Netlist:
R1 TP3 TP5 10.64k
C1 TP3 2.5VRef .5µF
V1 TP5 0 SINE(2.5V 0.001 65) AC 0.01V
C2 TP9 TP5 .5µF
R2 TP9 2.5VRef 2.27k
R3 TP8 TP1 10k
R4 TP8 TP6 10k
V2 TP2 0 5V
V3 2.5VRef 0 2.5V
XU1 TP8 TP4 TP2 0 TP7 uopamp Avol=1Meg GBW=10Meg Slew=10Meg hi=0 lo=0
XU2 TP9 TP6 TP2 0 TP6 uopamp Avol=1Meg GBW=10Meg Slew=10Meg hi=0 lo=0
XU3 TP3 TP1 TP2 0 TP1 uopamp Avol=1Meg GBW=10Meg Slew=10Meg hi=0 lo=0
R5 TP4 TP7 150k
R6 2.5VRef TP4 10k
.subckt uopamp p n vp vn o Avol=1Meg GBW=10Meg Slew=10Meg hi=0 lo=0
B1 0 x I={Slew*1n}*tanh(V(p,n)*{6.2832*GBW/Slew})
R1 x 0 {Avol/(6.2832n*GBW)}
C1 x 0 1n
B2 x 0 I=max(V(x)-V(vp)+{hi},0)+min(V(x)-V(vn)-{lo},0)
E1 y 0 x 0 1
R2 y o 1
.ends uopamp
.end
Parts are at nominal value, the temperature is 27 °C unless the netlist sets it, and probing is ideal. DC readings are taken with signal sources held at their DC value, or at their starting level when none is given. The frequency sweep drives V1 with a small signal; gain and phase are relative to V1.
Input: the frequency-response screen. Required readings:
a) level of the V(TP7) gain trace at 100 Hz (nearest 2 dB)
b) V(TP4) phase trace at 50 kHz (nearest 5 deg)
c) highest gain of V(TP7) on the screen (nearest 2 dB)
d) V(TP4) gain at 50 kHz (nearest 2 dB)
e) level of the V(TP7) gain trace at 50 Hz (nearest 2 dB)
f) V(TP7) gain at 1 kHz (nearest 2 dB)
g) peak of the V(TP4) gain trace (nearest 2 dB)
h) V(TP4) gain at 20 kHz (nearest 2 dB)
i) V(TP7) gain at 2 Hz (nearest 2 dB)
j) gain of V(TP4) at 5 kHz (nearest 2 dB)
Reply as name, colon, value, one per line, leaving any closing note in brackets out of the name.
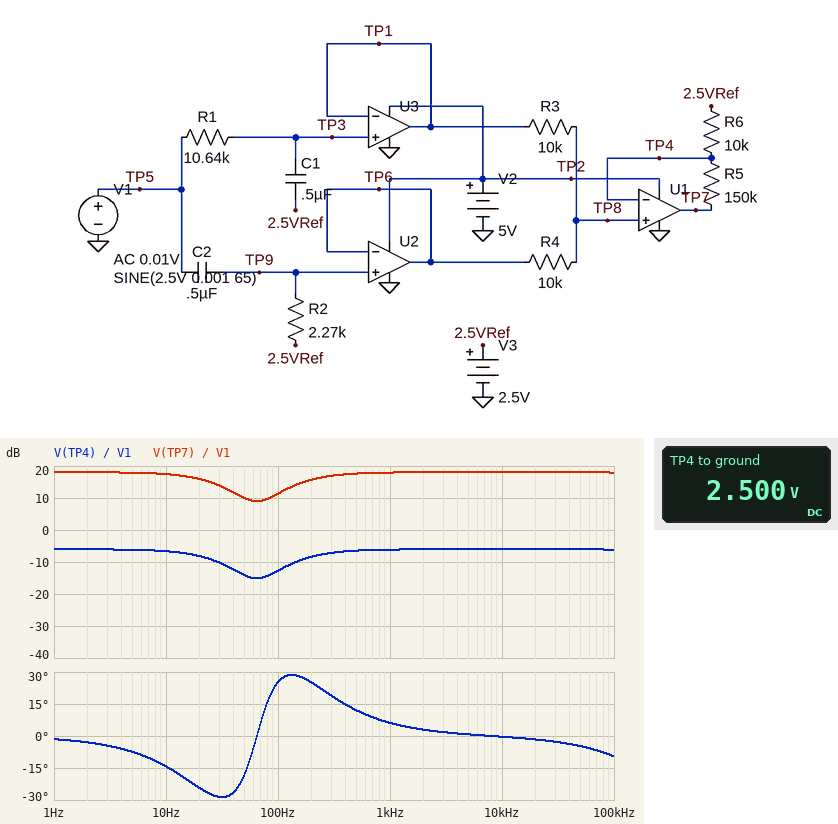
level of the V(TP7) gain trace at 100 Hz: 12 dB
V(TP4) phase trace at 50 kHz: -5 deg
highest gain of V(TP7) on the screen: 18 dB
V(TP4) gain at 50 kHz: -6 dB
level of the V(TP7) gain trace at 50 Hz: 10 dB
V(TP7) gain at 1 kHz: 18 dB
peak of the V(TP4) gain trace: -6 dB
V(TP4) gain at 20 kHz: -6 dB
V(TP7) gain at 2 Hz: 18 dB
gain of V(TP4) at 5 kHz: -6 dB
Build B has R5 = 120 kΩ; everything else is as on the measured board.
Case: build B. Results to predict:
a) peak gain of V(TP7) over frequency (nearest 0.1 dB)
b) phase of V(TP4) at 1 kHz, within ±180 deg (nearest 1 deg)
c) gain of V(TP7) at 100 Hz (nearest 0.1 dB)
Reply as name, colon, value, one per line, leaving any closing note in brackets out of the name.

peak gain of V(TP7) over frequency: 16.3 dB
phase of V(TP4) at 1 kHz, within ±180 deg: 6 deg
gain of V(TP7) at 100 Hz: 9.6 dB
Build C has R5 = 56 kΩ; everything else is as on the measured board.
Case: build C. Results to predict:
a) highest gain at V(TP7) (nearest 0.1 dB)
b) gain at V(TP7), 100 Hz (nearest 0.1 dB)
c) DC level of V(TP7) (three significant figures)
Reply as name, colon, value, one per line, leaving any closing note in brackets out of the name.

highest gain at V(TP7): 10.4 dB
gain at V(TP7), 100 Hz: 3.7 dB
DC level of V(TP7): 2.50 V
